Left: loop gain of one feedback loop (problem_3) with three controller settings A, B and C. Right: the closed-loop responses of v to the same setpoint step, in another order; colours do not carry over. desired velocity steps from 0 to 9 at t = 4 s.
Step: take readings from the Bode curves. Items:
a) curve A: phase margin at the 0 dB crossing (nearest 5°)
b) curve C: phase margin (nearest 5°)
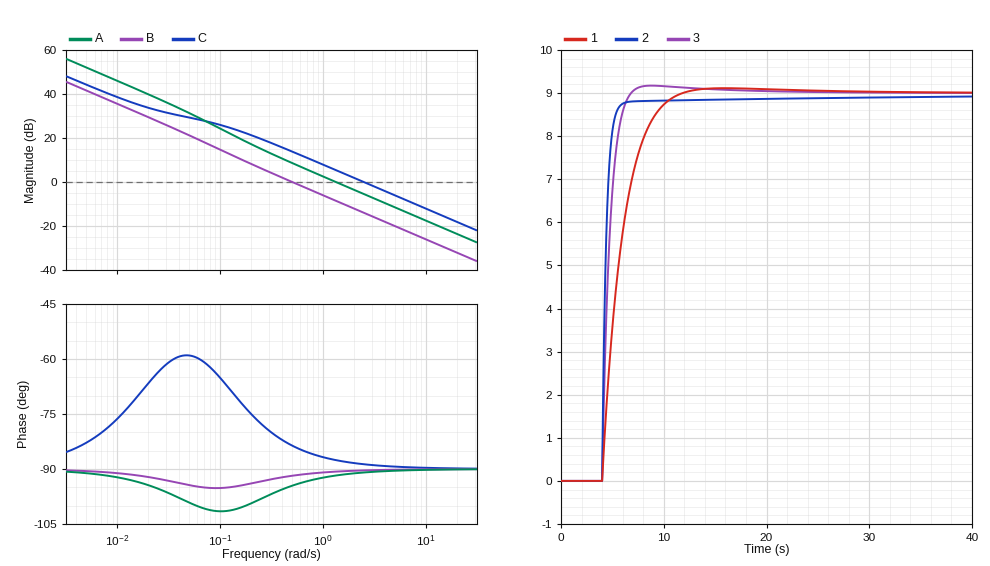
90°
90°
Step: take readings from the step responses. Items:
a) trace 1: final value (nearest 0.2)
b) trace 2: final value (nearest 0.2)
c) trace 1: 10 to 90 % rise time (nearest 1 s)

9.0
9.0
4 s
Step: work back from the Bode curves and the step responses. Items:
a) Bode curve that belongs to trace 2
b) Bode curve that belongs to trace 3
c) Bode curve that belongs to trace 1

C
A
B
